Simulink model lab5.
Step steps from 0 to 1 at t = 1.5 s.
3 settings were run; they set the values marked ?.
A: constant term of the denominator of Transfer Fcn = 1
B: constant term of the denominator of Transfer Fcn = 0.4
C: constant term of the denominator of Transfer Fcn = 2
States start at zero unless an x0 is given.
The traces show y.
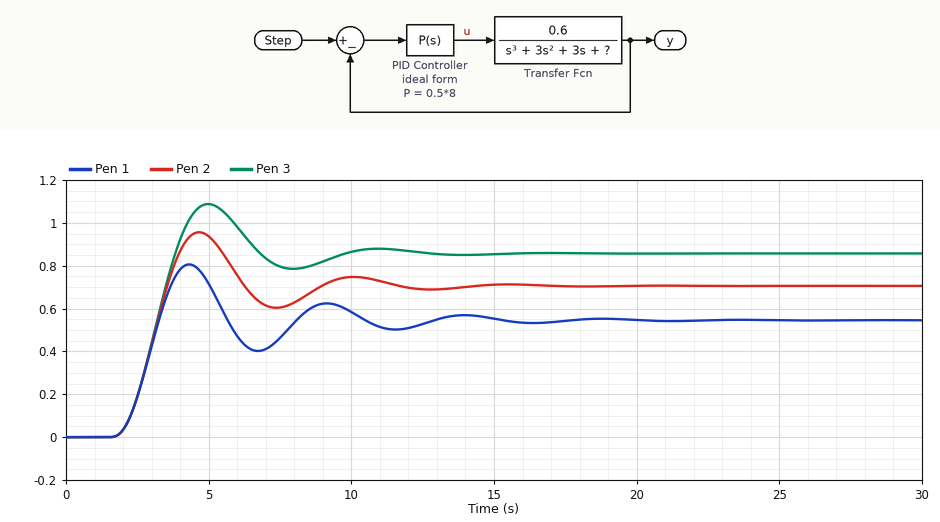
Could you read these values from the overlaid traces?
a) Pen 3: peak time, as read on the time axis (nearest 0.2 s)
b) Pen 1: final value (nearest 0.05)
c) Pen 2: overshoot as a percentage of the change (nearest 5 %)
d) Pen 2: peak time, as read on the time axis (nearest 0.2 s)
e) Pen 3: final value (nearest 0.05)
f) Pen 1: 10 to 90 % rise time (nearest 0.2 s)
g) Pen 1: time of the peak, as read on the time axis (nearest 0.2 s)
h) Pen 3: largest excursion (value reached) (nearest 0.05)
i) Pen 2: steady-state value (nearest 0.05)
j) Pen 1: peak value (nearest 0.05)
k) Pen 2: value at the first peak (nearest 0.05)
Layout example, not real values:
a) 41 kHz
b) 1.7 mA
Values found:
a) 5.0 s
b) 0.55
c) 35 %
d) 4.6 s
e) 0.85
f) 1.0 s
g) 4.4 s
h) 1.10
i) 0.70
j) 0.80
k) 0.95
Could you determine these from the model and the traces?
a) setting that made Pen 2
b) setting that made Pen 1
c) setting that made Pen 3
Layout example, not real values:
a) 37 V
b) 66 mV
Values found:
a) A
b) C
c) B
